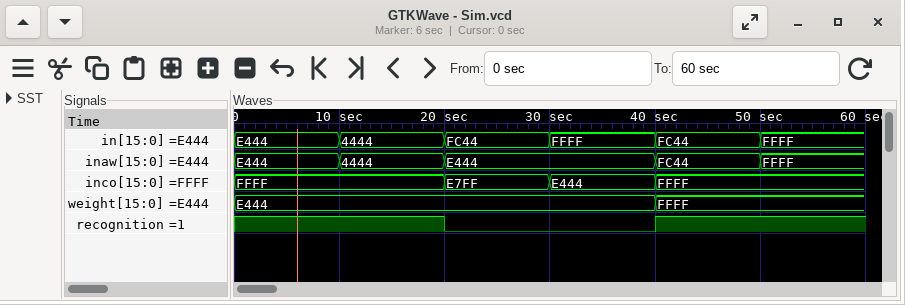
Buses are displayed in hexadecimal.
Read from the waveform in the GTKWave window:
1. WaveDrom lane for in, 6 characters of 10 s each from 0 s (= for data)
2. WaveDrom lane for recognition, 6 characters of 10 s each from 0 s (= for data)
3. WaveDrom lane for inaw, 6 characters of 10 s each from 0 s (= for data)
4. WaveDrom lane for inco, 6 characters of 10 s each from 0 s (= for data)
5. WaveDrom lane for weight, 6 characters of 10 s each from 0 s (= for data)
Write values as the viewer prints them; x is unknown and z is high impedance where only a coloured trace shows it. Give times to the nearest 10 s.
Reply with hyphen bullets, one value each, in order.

- {name: 'in', wave: '======', data: 'E444 4444 FC44 FFFF FC44 FFFF'}
- {name: 'recognition', wave: '1.0.1.'}
- {name: 'inaw', wave: '===.==', data: 'E444 4444 E444 FC44 FFFF'}
- {name: 'inco', wave: '=.===.', data: 'FFFF E7FF E444 FFFF'}
- {name: 'weight', wave: '=...=.', data: 'E444 FFFF'}
